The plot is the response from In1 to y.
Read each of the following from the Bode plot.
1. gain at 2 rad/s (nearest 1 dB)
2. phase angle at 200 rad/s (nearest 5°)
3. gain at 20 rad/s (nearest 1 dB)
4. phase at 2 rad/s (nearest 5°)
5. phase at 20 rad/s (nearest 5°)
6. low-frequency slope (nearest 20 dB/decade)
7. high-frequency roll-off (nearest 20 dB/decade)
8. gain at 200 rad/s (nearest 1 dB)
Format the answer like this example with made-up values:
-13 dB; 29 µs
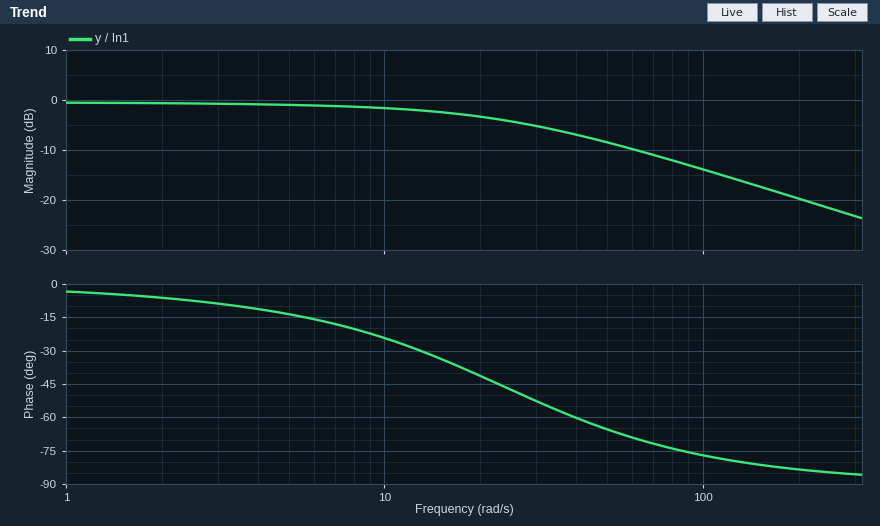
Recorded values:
-1 dB; -85°; -3 dB; -5°; -40°; 0 dB/decade; -20 dB/decade; -20 dB
